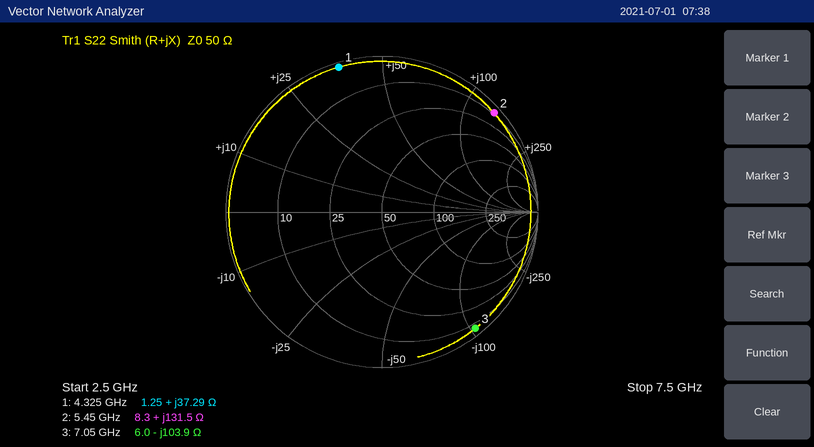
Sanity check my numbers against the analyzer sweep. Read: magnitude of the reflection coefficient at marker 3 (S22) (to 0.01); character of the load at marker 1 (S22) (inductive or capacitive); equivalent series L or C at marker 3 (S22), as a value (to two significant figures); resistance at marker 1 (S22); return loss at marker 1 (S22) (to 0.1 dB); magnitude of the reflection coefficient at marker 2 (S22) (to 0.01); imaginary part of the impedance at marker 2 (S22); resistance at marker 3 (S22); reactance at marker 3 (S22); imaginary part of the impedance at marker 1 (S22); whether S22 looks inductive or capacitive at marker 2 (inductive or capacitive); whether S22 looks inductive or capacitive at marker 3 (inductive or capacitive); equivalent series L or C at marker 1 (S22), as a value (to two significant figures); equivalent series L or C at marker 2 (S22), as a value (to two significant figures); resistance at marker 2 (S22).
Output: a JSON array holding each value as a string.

["0.96", "inductive", "220 fF", "1.25 Ω", "0.3 dB", "0.96", "+131.5 Ω", "6.0 Ω", "-103.9 Ω", "+37.29 Ω", "inductive", "capacitive", "1.4 nH", "3.8 nH", "8.3 Ω"]
